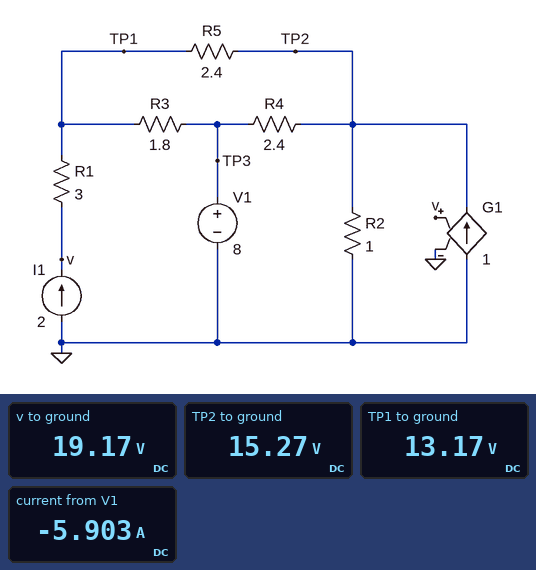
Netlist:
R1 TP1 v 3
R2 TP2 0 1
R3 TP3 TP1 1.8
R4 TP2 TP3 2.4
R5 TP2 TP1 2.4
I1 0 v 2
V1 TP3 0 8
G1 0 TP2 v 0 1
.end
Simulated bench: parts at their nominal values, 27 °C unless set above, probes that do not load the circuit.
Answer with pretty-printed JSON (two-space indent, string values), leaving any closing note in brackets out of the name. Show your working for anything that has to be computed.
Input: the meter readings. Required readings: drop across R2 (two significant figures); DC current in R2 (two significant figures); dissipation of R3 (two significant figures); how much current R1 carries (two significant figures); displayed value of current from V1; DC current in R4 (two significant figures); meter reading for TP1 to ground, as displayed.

{
  "drop across R2": "15.27 V = 15 V",
  "DC current in R2": "(15.27 V) / 1 Ω = 15 A",
  "dissipation of R3": "(13.17 V - 8 V)^2 / 1.8 Ω = 15 W",
  "how much current R1 carries": "(19.17 V - 13.17 V) / 3 Ω = 2.0 A",
  "displayed value of current from V1": "-5.903 A",
  "DC current in R4": "(15.27 V - 8 V) / 2.4 Ω = 3.0 A",
  "meter reading for TP1 to ground, as displayed": "13.17 V"
}
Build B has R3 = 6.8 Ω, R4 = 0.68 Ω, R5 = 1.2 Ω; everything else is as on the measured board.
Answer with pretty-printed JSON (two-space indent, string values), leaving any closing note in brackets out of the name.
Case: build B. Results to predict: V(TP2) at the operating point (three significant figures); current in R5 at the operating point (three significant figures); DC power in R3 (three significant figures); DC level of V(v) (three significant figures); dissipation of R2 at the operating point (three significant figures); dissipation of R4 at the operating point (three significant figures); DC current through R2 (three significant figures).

{
  "V(TP2) at the operating point": "13.6 V",
  "current in R5 at the operating point": "1.00 A",
  "DC power in R3": "6.77 W",
  "DC level of V(v)": "20.8 V",
  "dissipation of R2 at the operating point": "184 W",
  "dissipation of R4 at the operating point": "45.8 W",
  "DC current through R2": "13.6 A"
}
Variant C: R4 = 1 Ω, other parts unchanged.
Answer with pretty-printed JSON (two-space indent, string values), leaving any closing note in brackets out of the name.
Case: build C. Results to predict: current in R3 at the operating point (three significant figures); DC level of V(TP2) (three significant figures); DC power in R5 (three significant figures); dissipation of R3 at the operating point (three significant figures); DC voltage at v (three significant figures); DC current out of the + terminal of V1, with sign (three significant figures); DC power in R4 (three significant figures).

{
  "current in R3 at the operating point": "2.32 A",
  "DC level of V(TP2)": "12.9 V",
  "DC power in R5": "239 mW",
  "dissipation of R3 at the operating point": "9.65 W",
  "DC voltage at v": "18.2 V",
  "DC current out of the + terminal of V1, with sign": "-7.24 A",
  "DC power in R4": "24.3 W"
}
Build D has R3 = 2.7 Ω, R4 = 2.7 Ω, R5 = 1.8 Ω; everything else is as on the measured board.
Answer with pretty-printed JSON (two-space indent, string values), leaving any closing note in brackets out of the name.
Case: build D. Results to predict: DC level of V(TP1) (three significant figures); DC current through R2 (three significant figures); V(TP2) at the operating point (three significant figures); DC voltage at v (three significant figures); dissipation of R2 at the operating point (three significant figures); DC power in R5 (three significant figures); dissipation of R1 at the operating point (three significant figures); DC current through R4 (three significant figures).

{
  "DC level of V(TP1)": "15.8 V",
  "DC current through R2": "17.4 A",
  "V(TP2) at the operating point": "17.4 V",
  "DC voltage at v": "21.8 V",
  "dissipation of R2 at the operating point": "304 W",
  "DC power in R5": "1.44 W",
  "dissipation of R1 at the operating point": "12.0 W",
  "DC current through R4": "3.49 A"
}
